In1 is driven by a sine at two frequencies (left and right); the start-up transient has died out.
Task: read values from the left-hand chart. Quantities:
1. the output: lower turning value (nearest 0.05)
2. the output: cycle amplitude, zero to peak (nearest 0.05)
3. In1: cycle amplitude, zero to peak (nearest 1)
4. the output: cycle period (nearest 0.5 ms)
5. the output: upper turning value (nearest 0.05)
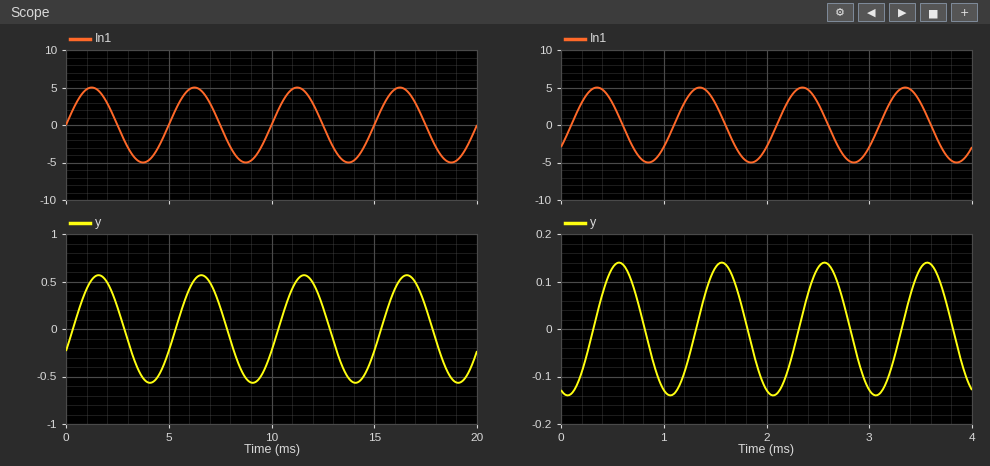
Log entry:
-0.55
0.55
5
5.0 ms
0.55
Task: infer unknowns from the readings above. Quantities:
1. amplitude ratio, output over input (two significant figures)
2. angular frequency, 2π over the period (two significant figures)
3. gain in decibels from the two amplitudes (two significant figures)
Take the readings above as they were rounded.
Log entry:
0.11
1.3 rad/ms
-19 dB
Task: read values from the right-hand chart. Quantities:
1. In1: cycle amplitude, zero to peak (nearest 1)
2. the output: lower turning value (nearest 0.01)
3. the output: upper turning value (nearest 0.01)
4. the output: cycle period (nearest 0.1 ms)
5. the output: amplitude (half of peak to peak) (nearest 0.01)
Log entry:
5
-0.14
0.14
1.0 ms
0.14
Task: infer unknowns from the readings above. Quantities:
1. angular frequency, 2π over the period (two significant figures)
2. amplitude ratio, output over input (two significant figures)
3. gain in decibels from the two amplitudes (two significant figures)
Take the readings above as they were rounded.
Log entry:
6.3 rad/ms
0.028
-31 dB
